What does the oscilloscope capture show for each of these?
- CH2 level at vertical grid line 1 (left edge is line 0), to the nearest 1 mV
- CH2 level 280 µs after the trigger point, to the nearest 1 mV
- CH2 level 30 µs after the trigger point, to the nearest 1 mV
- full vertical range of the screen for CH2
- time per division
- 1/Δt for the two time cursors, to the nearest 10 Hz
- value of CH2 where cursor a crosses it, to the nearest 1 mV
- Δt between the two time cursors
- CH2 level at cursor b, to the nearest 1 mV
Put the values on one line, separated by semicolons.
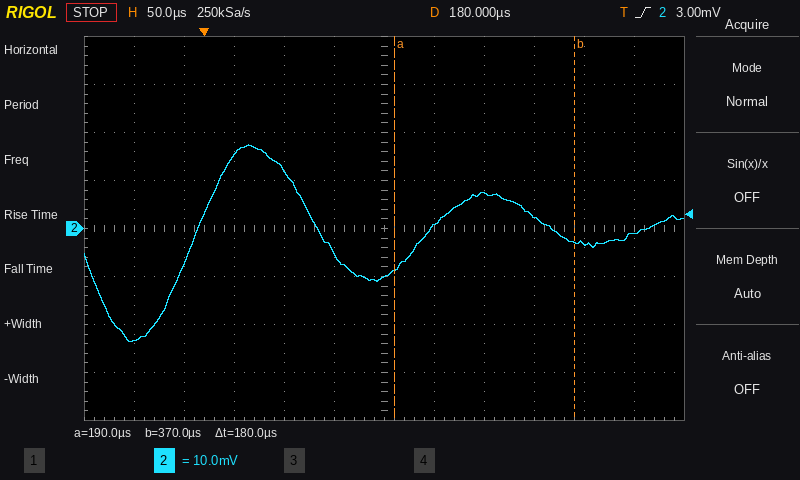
-23 mV; 7 mV; 15 mV; 80 mV; 50 µs; 5.56 kHz; -9 mV; 180 µs; -3 mV
